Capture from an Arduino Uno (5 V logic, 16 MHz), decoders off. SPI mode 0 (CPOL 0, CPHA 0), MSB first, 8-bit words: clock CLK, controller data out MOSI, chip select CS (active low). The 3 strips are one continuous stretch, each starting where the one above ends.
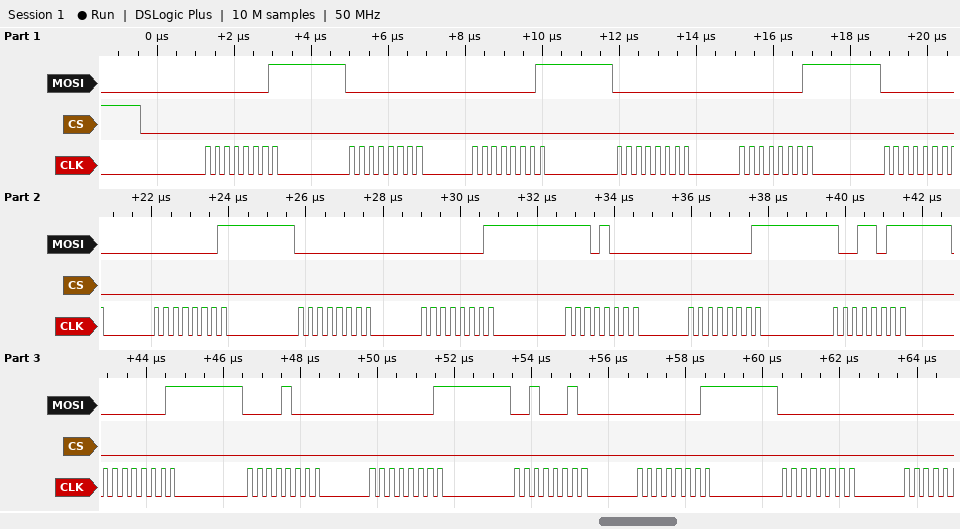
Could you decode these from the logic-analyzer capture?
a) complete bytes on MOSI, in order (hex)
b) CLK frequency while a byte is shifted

0x01 0x00 0x01 0x00 0x01 0x00 0x01 0x00 0x01 0xE8 0x01 0x9B 0x01 0x08 0x01 0x22 0x01 0x00
4 MHz
